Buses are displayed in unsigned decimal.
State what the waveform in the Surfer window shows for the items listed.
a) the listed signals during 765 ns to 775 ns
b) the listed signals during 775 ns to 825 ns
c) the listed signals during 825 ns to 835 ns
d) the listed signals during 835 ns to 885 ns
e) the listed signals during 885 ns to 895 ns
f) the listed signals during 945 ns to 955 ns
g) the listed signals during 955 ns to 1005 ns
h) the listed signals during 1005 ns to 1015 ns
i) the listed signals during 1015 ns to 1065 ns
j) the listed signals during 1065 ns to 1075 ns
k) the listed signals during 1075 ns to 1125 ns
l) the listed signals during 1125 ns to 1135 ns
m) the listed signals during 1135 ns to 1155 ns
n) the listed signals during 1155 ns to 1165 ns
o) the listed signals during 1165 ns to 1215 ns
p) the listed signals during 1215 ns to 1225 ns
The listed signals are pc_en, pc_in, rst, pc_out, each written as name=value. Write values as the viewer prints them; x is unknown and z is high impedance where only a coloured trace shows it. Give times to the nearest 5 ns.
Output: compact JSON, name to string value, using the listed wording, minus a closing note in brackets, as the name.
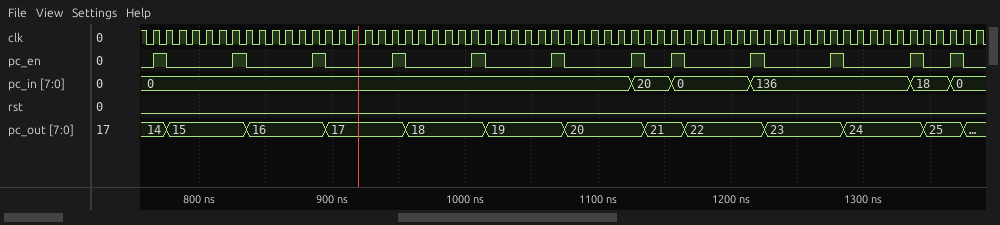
{"the listed signals during 765 ns to 775 ns": "pc_en=1, pc_in=0, rst=0, pc_out=14", "the listed signals during 775 ns to 825 ns": "pc_en=0, pc_in=0, rst=0, pc_out=15", "the listed signals during 825 ns to 835 ns": "pc_en=1, pc_in=0, rst=0, pc_out=15", "the listed signals during 835 ns to 885 ns": "pc_en=0, pc_in=0, rst=0, pc_out=16", "the listed signals during 885 ns to 895 ns": "pc_en=1, pc_in=0, rst=0, pc_out=16", "the listed signals during 945 ns to 955 ns": "pc_en=1, pc_in=0, rst=0, pc_out=17", "the listed signals during 955 ns to 1005 ns": "pc_en=0, pc_in=0, rst=0, pc_out=18", "the listed signals during 1005 ns to 1015 ns": "pc_en=1, pc_in=0, rst=0, pc_out=18", "the listed signals during 1015 ns to 1065 ns": "pc_en=0, pc_in=0, rst=0, pc_out=19", "the listed signals during 1065 ns to 1075 ns": "pc_en=1, pc_in=0, rst=0, pc_out=19", "the listed signals during 1075 ns to 1125 ns": "pc_en=0, pc_in=0, rst=0, pc_out=20", "the listed signals during 1125 ns to 1135 ns": "pc_en=1, pc_in=20, rst=0, pc_out=20", "the listed signals during 1135 ns to 1155 ns": "pc_en=0, pc_in=20, rst=0, pc_out=21", "the listed signals during 1155 ns to 1165 ns": "pc_en=1, pc_in=0, rst=0, pc_out=21", "the listed signals during 1165 ns to 1215 ns": "pc_en=0, pc_in=0, rst=0, pc_out=22", "the listed signals during 1215 ns to 1225 ns": "pc_en=1, pc_in=136, rst=0, pc_out=22"}
